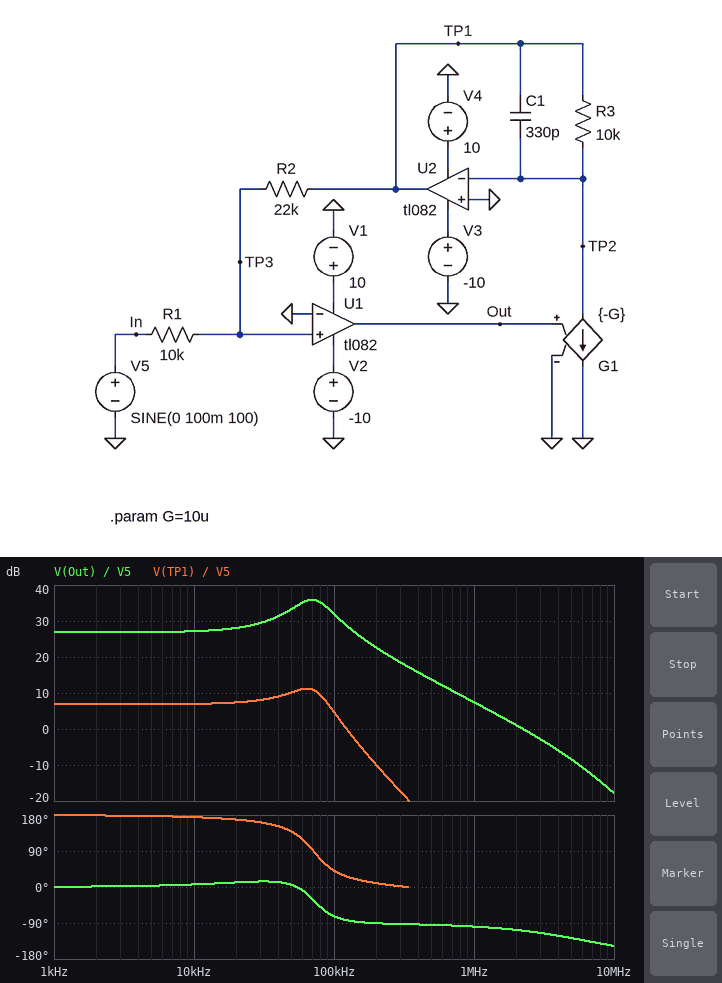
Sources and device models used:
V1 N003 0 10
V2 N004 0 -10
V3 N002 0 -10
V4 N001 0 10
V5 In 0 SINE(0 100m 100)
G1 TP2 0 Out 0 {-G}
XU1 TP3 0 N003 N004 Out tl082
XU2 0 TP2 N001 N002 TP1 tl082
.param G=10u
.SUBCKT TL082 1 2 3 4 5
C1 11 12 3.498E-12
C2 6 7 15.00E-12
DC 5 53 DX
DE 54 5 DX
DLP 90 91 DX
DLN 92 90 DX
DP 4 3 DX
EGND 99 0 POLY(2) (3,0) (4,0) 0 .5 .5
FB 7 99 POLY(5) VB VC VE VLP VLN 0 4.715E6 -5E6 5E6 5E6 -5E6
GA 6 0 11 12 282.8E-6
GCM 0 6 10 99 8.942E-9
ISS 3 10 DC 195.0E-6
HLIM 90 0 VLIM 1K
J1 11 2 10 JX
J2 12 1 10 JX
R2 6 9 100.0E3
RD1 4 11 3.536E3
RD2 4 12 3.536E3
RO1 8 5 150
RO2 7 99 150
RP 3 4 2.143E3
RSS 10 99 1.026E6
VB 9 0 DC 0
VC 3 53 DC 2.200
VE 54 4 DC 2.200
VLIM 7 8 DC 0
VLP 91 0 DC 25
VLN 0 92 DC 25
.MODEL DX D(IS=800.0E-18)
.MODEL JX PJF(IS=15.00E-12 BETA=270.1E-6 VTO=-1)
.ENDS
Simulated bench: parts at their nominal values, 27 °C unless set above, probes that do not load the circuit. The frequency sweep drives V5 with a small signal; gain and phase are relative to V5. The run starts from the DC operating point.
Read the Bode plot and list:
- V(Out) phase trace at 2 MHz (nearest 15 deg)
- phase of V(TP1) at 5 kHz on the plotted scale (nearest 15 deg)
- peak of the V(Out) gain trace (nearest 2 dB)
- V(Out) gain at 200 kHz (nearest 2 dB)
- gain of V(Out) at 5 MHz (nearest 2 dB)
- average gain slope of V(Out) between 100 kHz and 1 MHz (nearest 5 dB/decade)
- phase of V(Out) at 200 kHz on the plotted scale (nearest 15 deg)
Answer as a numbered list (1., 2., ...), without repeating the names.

1. -105 deg
2. 180 deg
3. 36 dB
4. 22 dB
5. -8 dB
6. -25 dB/decade
7. -90 deg
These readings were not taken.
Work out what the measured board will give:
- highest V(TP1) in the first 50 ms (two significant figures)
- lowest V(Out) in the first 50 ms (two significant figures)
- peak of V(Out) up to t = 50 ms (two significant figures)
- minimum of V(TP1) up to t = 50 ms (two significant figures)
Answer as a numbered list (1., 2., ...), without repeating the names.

1. 220 mV
2. -2.2 V
3. 2.2 V
4. -220 mV
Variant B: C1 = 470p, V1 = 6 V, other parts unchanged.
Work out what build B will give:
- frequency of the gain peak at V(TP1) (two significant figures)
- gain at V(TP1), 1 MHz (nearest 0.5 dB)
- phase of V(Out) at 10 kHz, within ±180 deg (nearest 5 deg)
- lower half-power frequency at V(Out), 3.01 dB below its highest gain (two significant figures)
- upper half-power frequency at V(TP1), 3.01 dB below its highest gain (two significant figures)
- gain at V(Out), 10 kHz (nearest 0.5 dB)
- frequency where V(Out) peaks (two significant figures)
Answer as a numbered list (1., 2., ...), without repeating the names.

1. 56 kHz
2. -41.0 dB
3. 10 deg
4. 44 kHz
5. 71 kHz
6. 27.5 dB
7. 59 kHz
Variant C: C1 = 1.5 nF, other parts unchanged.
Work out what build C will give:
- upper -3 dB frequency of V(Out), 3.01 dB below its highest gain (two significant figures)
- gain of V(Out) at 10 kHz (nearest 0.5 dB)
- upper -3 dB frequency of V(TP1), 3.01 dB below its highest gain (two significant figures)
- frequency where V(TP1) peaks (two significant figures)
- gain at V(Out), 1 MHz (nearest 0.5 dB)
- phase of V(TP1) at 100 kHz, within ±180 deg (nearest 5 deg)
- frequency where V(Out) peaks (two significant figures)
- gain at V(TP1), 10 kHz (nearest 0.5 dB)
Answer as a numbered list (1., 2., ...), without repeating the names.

1. 39 kHz
2. 30.5 dB
3. 38 kHz
4. 33 kHz
5. 7.5 dB
6. 5 deg
7. 34 kHz
8. 7.5 dB
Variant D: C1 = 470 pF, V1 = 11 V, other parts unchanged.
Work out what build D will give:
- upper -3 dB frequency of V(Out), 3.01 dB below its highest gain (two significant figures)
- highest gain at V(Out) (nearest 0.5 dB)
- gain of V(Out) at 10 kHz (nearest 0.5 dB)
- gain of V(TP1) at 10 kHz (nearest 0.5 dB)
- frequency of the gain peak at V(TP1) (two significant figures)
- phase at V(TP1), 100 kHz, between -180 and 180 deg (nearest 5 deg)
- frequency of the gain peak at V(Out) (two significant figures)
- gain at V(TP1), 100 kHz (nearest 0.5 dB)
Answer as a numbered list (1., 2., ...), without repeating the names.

1. 77 kHz
2. 38.5 dB
3. 27.5 dB
4. 7.0 dB
5. 56 kHz
6. 25 deg
7. 59 kHz
8. 1.0 dB
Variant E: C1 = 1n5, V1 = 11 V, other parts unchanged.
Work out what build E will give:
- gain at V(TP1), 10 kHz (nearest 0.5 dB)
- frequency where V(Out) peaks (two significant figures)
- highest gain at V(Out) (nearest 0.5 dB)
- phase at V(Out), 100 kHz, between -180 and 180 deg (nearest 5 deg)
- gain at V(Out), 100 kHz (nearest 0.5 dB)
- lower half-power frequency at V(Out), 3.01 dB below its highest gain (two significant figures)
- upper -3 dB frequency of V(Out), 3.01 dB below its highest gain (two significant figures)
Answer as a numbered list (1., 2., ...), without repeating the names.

1. 7.5 dB
2. 34 kHz
3. 48.0 dB
4. -90 deg
5. 28.5 dB
6. 29 kHz
7. 39 kHz
